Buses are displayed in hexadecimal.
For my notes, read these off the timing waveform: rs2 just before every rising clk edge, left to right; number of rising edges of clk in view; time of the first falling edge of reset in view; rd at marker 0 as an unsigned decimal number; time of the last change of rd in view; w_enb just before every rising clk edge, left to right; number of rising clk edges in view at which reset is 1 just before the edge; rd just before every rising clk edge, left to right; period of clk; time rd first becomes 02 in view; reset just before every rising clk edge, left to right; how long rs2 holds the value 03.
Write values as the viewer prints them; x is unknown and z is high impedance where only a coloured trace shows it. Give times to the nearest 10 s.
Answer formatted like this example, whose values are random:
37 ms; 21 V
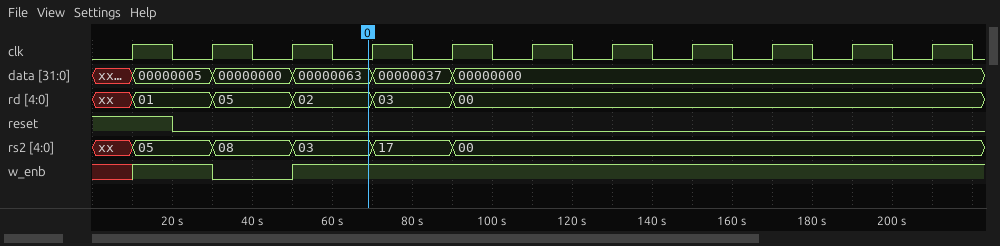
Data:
xx, 05, 08, 03, 17, 00, 00, 00, 00, 00, 00; 11; 20 s; 2; 90 s; x 1 0 1 1 1 1 1 1 1 1; 1; xx, 01, 05, 02, 03, 00, 00, 00, 00, 00, 00; 20 s; 50 s; 1 0 0 0 0 0 0 0 0 0 0; 20 s
